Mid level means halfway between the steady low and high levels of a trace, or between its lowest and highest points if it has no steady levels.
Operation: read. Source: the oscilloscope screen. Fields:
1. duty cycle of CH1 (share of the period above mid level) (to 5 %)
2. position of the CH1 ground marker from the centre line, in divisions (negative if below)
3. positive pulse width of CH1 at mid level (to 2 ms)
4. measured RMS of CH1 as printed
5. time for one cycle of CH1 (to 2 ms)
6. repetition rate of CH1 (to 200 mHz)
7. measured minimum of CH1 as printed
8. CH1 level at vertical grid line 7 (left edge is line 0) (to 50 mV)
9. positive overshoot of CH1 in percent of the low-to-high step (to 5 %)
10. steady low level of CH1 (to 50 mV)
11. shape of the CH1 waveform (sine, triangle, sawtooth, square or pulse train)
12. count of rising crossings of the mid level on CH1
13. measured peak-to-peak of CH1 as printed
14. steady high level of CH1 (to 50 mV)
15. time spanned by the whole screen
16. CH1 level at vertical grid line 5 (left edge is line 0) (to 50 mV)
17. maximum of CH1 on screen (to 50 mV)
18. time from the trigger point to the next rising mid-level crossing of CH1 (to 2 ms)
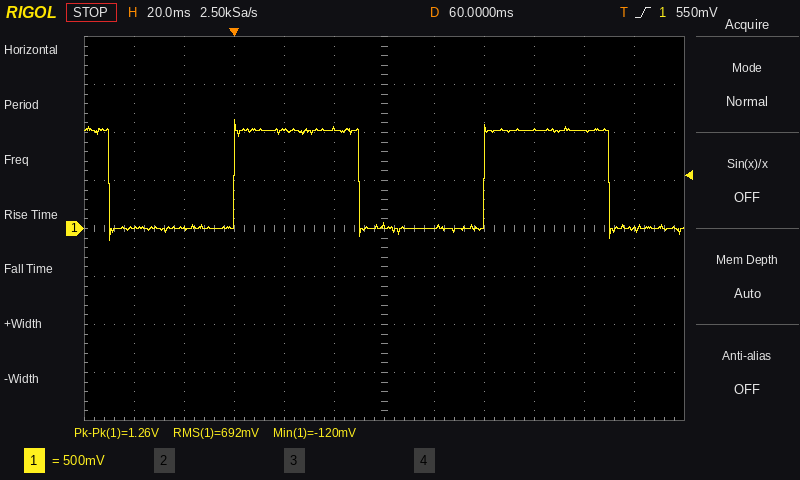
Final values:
50 %
0.0 div
50 ms
692 mV
100 ms
10.0 Hz
-120 mV
0 mV
10 %
0 mV
square
2
1.26 V
1.00 V
240 ms
1.05 V
1.15 V
100 ms
